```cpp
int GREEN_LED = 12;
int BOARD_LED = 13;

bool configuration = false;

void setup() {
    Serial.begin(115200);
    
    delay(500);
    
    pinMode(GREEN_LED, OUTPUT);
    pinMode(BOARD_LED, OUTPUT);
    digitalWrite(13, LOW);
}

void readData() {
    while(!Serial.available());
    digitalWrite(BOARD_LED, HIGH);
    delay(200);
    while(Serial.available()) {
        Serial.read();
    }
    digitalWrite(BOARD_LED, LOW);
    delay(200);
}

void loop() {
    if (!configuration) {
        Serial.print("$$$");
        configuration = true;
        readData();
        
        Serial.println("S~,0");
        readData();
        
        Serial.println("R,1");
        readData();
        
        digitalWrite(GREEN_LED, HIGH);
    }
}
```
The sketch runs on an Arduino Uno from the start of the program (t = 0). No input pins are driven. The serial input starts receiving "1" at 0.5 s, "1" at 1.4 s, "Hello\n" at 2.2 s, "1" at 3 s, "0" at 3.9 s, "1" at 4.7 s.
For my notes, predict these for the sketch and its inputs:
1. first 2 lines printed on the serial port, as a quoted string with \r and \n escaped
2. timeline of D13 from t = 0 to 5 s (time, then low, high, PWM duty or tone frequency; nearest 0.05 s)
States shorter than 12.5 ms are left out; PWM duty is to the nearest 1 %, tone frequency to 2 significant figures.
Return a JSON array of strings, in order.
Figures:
["\"$$$S~,0\\r\\nR,1\\r\\n\"", "0.5 s high; 0.7 s low; 1.4 s high; 1.6 s low; 2.2 s high; 2.4 s low"]
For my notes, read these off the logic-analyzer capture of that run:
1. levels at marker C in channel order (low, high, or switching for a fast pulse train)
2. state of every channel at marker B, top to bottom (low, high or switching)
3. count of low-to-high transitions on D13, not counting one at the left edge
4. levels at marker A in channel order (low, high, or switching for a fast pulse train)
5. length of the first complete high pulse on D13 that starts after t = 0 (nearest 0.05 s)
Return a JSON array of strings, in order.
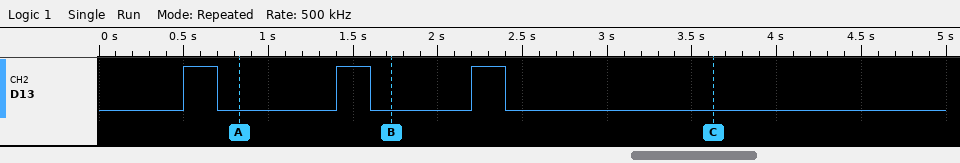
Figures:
["D13 low", "D13 low", "3", "D13 low", "0.20 s"]
